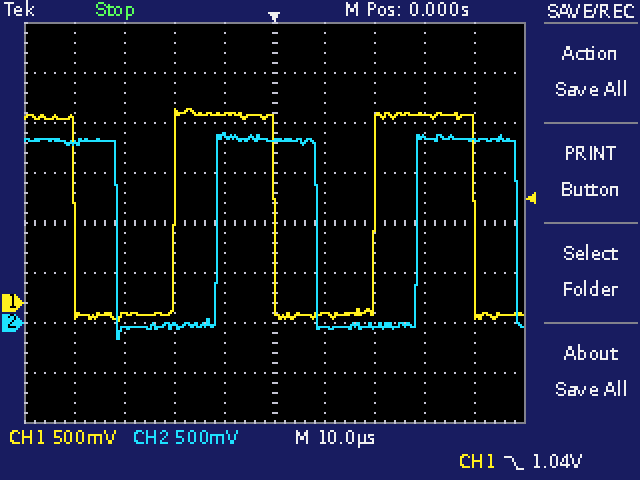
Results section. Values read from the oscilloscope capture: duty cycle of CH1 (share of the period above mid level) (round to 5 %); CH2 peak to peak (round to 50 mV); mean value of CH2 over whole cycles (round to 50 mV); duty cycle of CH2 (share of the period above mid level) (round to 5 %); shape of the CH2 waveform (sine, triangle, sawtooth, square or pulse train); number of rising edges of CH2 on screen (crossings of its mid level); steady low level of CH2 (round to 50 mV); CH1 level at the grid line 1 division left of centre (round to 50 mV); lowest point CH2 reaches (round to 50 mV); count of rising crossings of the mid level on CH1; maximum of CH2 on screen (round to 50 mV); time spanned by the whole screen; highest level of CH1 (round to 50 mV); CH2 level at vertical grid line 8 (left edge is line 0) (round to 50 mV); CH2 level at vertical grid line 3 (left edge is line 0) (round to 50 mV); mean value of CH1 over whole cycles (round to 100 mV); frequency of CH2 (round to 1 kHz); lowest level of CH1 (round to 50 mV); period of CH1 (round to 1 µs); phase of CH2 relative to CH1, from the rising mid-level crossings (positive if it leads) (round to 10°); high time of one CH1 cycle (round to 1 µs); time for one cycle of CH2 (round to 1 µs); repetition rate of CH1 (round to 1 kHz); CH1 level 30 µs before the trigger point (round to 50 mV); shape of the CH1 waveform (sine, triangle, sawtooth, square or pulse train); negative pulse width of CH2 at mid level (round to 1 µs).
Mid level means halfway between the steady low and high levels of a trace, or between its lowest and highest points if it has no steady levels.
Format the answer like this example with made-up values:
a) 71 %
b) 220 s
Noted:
a) 50 %
b) 2.05 V
c) 900 mV
d) 50 %
e) square
f) 2
g) -50 mV
h) 1.90 V
i) -150 mV
j) 2
k) 1.90 V
l) 100 µs
m) 1.95 V
n) 1.85 V
o) -50 mV
p) 900 mV
q) 25 kHz
r) -200 mV
s) 40 µs
t) -80°
u) 20 µs
v) 40 µs
w) 25 kHz
x) -100 mV
y) square
z) 20 µs
